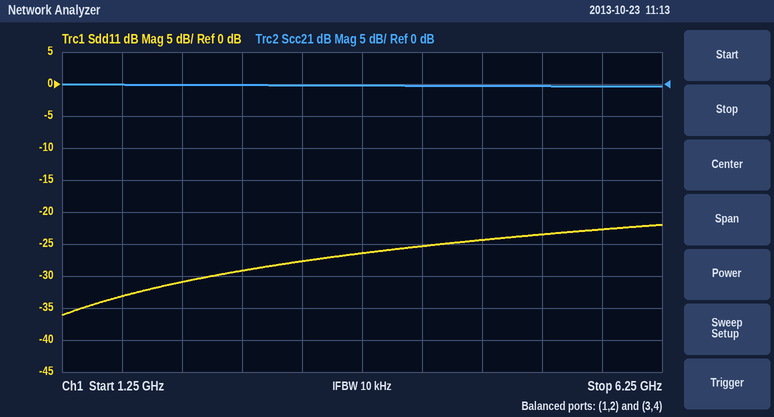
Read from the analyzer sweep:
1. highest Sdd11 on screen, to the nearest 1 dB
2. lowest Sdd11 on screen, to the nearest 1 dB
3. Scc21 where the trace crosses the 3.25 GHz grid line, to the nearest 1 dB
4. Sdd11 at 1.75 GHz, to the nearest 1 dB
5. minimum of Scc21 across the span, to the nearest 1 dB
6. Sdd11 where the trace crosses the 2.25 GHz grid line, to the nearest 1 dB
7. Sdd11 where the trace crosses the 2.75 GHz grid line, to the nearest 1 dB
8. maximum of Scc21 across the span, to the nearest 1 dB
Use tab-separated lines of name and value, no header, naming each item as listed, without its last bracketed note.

highest Sdd11 on screen, to the nearest 1 dB	-22 dB
lowest Sdd11 on screen, to the nearest 1 dB	-36 dB
Scc21 where the trace crosses the 3.25 GHz grid line, to the nearest 1 dB	0 dB
Sdd11 at 1.75 GHz, to the nearest 1 dB	-33 dB
minimum of Scc21 across the span, to the nearest 1 dB	0 dB
Sdd11 where the trace crosses the 2.25 GHz grid line, to the nearest 1 dB	-31 dB
Sdd11 where the trace crosses the 2.75 GHz grid line, to the nearest 1 dB	-29 dB
maximum of Scc21 across the span, to the nearest 1 dB	0 dB
